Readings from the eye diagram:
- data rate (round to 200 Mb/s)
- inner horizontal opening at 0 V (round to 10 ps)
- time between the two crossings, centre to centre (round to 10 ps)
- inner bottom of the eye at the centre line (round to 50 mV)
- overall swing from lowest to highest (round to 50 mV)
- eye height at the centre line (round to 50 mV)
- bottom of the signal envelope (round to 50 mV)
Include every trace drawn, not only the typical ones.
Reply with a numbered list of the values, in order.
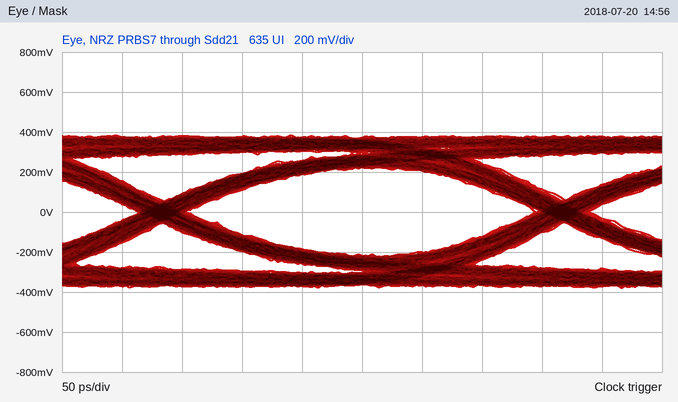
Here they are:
1. 3.0 Gb/s
2. 290 ps
3. 330 ps
4. -200 mV
5. 750 mV
6. 450 mV
7. -400 mV
